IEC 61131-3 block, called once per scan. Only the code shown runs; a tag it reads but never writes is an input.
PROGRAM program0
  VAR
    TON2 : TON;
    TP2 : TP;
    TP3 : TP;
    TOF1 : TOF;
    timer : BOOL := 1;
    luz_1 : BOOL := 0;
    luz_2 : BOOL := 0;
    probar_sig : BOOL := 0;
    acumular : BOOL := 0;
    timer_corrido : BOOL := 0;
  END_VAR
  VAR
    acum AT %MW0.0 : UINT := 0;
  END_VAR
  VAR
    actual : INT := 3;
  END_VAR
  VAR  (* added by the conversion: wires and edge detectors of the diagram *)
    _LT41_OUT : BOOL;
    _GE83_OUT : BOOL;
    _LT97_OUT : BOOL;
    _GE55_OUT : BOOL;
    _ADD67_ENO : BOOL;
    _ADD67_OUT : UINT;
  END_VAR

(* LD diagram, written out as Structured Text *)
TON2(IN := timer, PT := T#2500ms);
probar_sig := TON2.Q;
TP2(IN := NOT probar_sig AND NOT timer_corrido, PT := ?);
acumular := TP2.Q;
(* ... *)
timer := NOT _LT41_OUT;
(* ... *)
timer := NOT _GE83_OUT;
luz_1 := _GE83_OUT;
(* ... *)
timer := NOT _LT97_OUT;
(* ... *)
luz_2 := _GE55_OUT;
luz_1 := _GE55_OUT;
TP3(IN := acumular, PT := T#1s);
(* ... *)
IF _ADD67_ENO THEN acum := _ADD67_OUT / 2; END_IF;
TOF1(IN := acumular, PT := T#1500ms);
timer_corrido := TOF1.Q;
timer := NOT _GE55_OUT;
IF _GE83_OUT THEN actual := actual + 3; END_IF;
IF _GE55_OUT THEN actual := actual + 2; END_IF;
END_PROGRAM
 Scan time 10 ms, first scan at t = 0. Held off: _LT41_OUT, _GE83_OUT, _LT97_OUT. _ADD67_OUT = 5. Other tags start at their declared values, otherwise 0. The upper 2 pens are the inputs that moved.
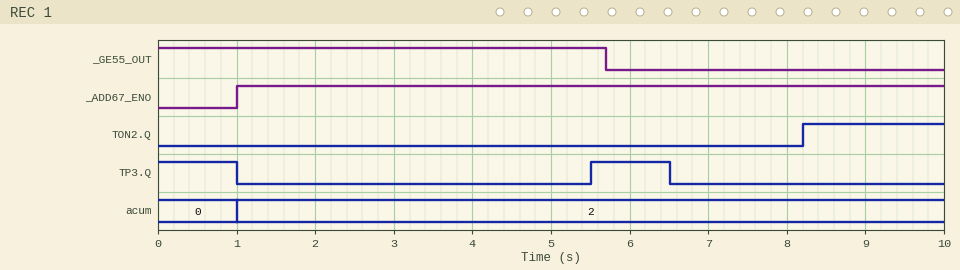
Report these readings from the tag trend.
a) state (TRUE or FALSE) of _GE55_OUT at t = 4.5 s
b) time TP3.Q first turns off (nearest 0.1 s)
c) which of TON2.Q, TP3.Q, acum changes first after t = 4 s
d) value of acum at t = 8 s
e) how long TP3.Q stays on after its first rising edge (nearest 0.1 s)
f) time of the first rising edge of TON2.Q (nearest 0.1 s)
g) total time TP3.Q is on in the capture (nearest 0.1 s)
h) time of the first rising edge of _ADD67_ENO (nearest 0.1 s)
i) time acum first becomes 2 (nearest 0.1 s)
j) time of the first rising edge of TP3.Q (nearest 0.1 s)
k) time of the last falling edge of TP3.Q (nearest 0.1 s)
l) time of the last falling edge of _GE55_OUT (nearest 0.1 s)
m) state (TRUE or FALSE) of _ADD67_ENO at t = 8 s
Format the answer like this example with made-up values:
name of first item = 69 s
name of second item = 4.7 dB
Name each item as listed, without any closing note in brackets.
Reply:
state (TRUE or FALSE) of _GE55_OUT at t = 4.5 s = TRUE
time TP3.Q first turns off = 1.0 s
which of TON2.Q, TP3.Q, acum changes first after t = 4 s = TP3.Q
value of acum at t = 8 s = 2
how long TP3.Q stays on after its first rising edge = 1.0 s
time of the first rising edge of TON2.Q = 8.2 s
total time TP3.Q is on in the capture = 2.0 s
time of the first rising edge of _ADD67_ENO = 1.0 s
time acum first becomes 2 = 1.0 s
time of the first rising edge of TP3.Q = 5.5 s
time of the last falling edge of TP3.Q = 6.5 s
time of the last falling edge of _GE55_OUT = 5.7 s
state (TRUE or FALSE) of _ADD67_ENO at t = 8 s = TRUE
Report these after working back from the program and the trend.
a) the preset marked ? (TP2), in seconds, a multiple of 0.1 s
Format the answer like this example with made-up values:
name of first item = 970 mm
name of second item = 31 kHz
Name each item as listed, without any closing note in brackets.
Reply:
the preset marked ? (TP2), in seconds, a multiple of 0.1 s = 4.0 s
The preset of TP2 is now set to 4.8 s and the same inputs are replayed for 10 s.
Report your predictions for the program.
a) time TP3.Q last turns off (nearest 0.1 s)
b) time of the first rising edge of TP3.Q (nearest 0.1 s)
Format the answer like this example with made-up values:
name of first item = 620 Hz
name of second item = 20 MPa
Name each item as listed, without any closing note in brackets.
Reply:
time TP3.Q last turns off = 7.3 s
time of the first rising edge of TP3.Q = 6.3 s
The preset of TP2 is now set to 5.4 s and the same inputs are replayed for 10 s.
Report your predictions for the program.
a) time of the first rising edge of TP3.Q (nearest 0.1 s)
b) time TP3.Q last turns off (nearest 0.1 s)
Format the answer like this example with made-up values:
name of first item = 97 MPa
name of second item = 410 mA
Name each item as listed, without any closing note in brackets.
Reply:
time of the first rising edge of TP3.Q = 6.9 s
time TP3.Q last turns off = 7.9 s
